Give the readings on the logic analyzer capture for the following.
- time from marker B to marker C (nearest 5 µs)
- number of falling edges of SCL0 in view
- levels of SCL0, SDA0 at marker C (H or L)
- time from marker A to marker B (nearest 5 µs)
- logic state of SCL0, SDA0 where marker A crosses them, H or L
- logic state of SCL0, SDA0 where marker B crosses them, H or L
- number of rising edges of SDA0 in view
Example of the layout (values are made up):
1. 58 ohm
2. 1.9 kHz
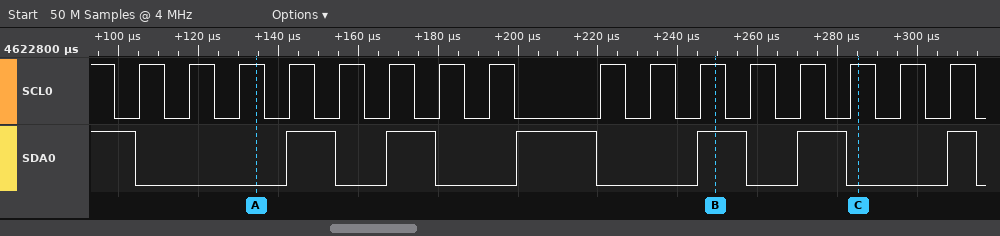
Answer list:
1. 35 µs
2. 17
3. SCL0=H, SDA0=L
4. 115 µs
5. SCL0=H, SDA0=L
6. SCL0=H, SDA0=H
7. 6
